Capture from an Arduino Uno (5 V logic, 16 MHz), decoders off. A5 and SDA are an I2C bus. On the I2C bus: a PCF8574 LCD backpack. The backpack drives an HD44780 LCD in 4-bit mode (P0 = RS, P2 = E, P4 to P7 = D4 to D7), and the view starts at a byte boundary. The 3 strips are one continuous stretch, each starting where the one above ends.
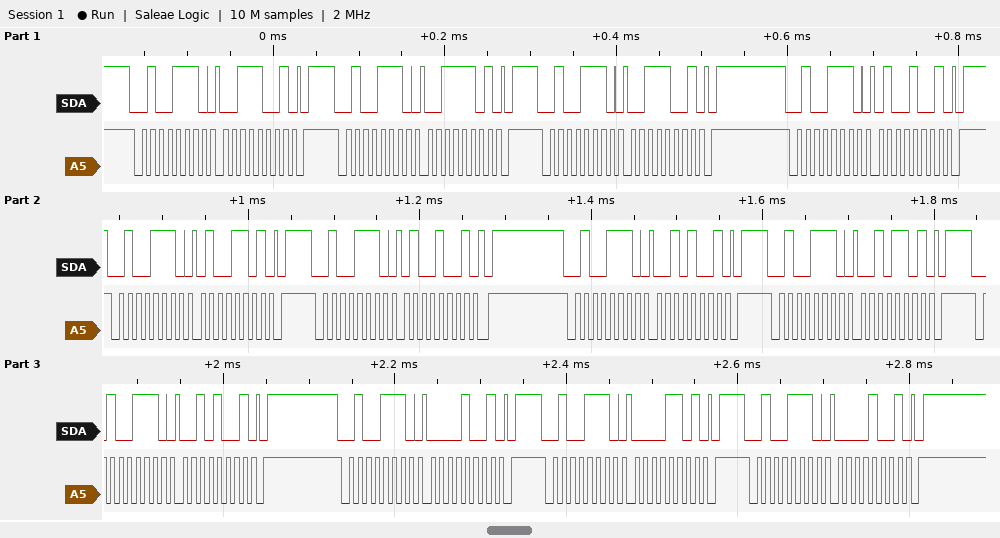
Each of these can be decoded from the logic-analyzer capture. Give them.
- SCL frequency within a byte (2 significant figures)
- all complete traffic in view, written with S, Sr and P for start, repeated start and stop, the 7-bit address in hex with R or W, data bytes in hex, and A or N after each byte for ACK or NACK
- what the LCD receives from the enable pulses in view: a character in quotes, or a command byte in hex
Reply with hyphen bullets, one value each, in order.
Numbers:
- 100 kHz
- S 27W A 39 A P S 27W A 3D A P S 27W A 39 A P S 27W A 49 A P S 27W A 4D A P S 27W A 49 A P S 27W A 29 A P S 27W A 2D A P S 27W A 29 A P S 27W A 09 A P S 27W A 0D A P S 27W A 09 A P
- '4' ' '
